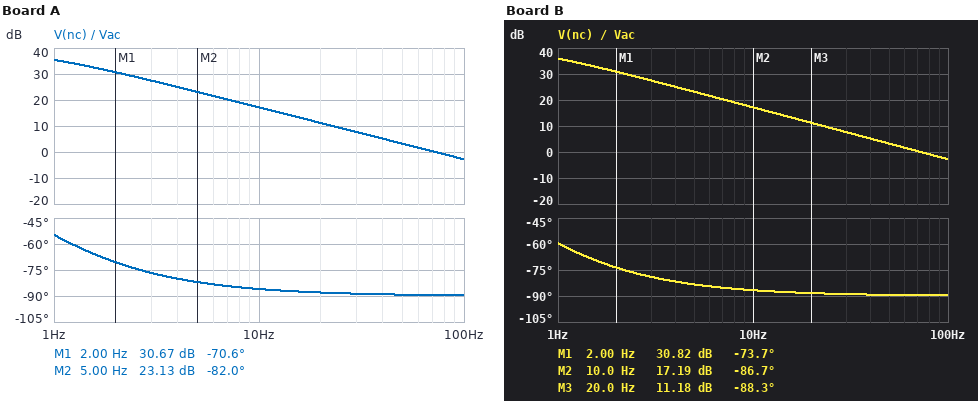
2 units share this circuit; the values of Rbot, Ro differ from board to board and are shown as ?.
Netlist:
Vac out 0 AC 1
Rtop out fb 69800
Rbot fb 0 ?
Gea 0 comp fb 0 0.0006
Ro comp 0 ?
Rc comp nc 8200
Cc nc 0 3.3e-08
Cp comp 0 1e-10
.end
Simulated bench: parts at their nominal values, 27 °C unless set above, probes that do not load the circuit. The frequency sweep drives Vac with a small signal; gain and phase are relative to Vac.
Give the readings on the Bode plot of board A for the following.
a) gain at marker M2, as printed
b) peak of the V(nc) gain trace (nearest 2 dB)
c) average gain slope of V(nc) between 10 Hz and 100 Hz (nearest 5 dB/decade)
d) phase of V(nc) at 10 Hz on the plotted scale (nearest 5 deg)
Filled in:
23.13 dB
36 dB
-20 dB/decade
-85 deg
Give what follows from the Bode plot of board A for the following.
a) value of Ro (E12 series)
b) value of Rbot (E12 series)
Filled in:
6.8 MΩ
1.8 kΩ
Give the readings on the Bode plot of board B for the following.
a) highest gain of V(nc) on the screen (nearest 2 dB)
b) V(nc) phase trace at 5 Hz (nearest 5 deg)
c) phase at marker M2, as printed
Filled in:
36 dB
-85 deg
-86.7 deg
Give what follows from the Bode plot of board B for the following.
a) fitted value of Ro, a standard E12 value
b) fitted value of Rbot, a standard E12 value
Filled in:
8.2 MΩ
1.8 kΩ
